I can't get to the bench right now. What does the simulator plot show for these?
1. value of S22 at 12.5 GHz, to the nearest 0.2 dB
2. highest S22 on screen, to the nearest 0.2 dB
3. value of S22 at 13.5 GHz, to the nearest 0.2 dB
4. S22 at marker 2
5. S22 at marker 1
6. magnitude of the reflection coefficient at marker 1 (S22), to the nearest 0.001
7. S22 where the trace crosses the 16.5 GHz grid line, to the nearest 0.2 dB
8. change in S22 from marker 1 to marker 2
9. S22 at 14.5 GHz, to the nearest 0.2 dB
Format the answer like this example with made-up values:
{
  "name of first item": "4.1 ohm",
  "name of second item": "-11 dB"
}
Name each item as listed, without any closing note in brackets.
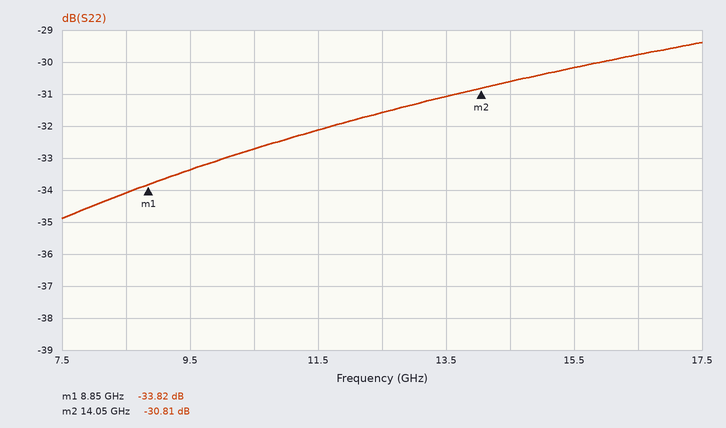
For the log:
{
  "value of S22 at 12.5 GHz, to the nearest 0.2 dB": "-31.6 dB",
  "highest S22 on screen, to the nearest 0.2 dB": "-29.4 dB",
  "value of S22 at 13.5 GHz, to the nearest 0.2 dB": "-31.0 dB",
  "S22 at marker 2": "-30.81 dB",
  "S22 at marker 1": "-33.82 dB",
  "magnitude of the reflection coefficient at marker 1 (S22), to the nearest 0.001": "0.020",
  "S22 where the trace crosses the 16.5 GHz grid line, to the nearest 0.2 dB": "-29.8 dB",
  "change in S22 from marker 1 to marker 2": "3.01 dB",
  "S22 at 14.5 GHz, to the nearest 0.2 dB": "-30.6 dB"
}
